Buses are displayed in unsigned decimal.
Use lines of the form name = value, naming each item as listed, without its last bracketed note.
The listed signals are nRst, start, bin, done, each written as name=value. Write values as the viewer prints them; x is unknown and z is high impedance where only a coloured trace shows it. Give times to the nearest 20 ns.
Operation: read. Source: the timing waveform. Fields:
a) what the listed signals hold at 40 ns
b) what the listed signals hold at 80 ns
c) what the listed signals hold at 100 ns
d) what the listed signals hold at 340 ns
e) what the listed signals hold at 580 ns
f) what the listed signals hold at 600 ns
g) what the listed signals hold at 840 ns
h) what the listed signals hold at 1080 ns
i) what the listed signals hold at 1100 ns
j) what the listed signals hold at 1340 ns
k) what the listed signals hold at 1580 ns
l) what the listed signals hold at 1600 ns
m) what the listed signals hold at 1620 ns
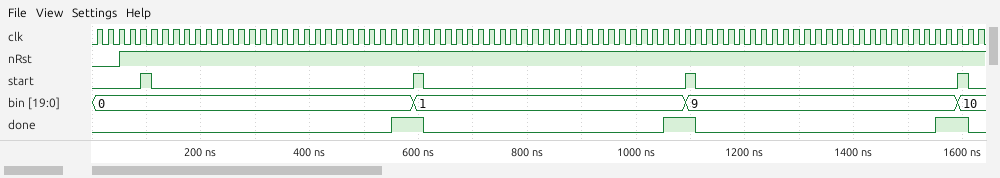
what the listed signals hold at 40 ns = nRst=0, start=0, bin=0, done=0
what the listed signals hold at 80 ns = nRst=1, start=0, bin=0, done=0
what the listed signals hold at 100 ns = nRst=1, start=1, bin=0, done=0
what the listed signals hold at 340 ns = nRst=1, start=0, bin=0, done=0
what the listed signals hold at 580 ns = nRst=1, start=0, bin=0, done=1
what the listed signals hold at 600 ns = nRst=1, start=1, bin=1, done=1
what the listed signals hold at 840 ns = nRst=1, start=0, bin=1, done=0
what the listed signals hold at 1080 ns = nRst=1, start=0, bin=1, done=1
what the listed signals hold at 1100 ns = nRst=1, start=1, bin=9, done=1
what the listed signals hold at 1340 ns = nRst=1, start=0, bin=9, done=0
what the listed signals hold at 1580 ns = nRst=1, start=0, bin=9, done=1
what the listed signals hold at 1600 ns = nRst=1, start=1, bin=10, done=1
what the listed signals hold at 1620 ns = nRst=1, start=0, bin=10, done=0
